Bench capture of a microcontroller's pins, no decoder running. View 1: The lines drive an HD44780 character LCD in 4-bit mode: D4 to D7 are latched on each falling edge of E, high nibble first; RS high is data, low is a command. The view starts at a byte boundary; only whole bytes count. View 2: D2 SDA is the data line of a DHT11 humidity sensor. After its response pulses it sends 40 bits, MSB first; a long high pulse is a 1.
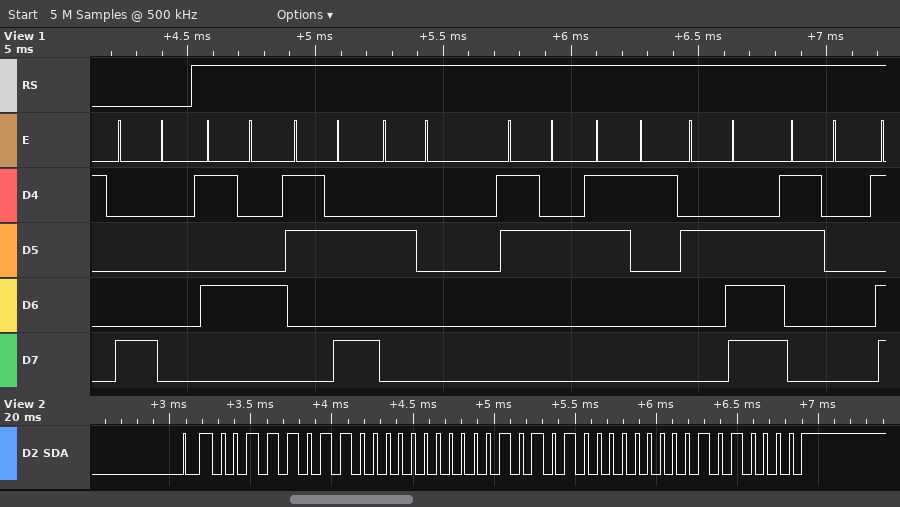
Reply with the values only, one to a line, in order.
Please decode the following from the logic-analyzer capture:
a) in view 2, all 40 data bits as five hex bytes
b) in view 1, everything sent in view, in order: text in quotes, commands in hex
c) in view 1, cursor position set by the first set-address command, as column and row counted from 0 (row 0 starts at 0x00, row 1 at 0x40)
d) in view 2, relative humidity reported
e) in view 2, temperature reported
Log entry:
3B 00 15 00 50
0x80 "T: 21.0"
column 0, row 0
59 %
21.0 °C
